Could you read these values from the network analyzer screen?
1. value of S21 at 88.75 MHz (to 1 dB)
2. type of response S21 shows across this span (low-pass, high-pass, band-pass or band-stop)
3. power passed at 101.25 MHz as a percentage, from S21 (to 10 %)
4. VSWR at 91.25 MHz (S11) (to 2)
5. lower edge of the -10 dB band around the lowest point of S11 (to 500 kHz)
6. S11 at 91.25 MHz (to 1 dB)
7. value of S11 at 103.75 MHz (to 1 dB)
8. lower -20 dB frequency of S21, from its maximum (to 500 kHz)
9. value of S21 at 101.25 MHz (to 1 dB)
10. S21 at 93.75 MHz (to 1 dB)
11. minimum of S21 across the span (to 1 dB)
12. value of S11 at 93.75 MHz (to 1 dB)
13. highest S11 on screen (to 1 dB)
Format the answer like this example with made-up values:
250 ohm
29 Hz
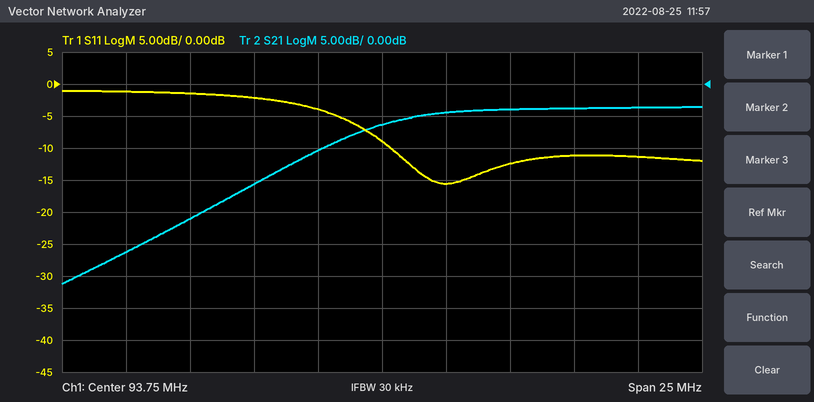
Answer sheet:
-16 dB
high-pass
40 %
4
94.0 MHz
-4 dB
-11 dB
85.0 MHz
-4 dB
-6 dB
-31 dB
-9 dB
-1 dB
